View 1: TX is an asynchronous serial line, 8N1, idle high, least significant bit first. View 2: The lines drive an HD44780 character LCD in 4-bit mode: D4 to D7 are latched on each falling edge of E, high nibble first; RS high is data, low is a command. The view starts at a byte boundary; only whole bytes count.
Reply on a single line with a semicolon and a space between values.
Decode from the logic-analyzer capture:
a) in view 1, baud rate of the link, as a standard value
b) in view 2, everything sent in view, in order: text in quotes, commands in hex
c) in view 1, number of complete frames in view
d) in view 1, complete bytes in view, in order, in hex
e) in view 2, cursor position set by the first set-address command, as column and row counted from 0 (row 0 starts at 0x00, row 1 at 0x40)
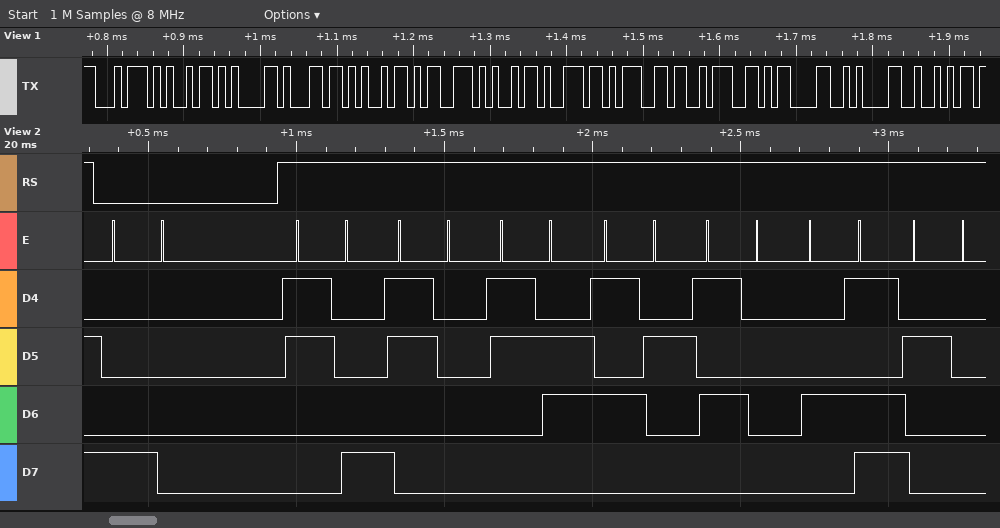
115200 baud; 0x80 "806RPM "; 13; 0x74 0x69 0x61 0x6C 0x69 0x73 0x69 0x6E 0x67 0x3A 0x0D 0x0A 0x52; column 0, row 0
